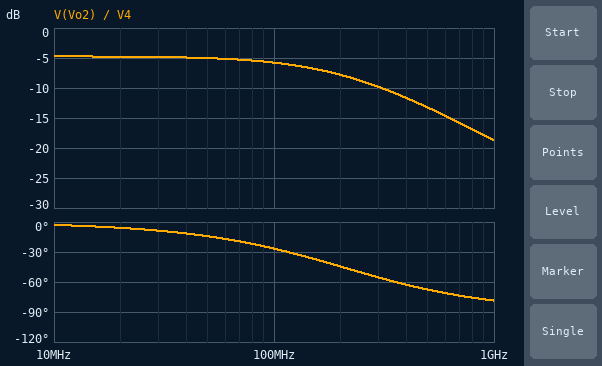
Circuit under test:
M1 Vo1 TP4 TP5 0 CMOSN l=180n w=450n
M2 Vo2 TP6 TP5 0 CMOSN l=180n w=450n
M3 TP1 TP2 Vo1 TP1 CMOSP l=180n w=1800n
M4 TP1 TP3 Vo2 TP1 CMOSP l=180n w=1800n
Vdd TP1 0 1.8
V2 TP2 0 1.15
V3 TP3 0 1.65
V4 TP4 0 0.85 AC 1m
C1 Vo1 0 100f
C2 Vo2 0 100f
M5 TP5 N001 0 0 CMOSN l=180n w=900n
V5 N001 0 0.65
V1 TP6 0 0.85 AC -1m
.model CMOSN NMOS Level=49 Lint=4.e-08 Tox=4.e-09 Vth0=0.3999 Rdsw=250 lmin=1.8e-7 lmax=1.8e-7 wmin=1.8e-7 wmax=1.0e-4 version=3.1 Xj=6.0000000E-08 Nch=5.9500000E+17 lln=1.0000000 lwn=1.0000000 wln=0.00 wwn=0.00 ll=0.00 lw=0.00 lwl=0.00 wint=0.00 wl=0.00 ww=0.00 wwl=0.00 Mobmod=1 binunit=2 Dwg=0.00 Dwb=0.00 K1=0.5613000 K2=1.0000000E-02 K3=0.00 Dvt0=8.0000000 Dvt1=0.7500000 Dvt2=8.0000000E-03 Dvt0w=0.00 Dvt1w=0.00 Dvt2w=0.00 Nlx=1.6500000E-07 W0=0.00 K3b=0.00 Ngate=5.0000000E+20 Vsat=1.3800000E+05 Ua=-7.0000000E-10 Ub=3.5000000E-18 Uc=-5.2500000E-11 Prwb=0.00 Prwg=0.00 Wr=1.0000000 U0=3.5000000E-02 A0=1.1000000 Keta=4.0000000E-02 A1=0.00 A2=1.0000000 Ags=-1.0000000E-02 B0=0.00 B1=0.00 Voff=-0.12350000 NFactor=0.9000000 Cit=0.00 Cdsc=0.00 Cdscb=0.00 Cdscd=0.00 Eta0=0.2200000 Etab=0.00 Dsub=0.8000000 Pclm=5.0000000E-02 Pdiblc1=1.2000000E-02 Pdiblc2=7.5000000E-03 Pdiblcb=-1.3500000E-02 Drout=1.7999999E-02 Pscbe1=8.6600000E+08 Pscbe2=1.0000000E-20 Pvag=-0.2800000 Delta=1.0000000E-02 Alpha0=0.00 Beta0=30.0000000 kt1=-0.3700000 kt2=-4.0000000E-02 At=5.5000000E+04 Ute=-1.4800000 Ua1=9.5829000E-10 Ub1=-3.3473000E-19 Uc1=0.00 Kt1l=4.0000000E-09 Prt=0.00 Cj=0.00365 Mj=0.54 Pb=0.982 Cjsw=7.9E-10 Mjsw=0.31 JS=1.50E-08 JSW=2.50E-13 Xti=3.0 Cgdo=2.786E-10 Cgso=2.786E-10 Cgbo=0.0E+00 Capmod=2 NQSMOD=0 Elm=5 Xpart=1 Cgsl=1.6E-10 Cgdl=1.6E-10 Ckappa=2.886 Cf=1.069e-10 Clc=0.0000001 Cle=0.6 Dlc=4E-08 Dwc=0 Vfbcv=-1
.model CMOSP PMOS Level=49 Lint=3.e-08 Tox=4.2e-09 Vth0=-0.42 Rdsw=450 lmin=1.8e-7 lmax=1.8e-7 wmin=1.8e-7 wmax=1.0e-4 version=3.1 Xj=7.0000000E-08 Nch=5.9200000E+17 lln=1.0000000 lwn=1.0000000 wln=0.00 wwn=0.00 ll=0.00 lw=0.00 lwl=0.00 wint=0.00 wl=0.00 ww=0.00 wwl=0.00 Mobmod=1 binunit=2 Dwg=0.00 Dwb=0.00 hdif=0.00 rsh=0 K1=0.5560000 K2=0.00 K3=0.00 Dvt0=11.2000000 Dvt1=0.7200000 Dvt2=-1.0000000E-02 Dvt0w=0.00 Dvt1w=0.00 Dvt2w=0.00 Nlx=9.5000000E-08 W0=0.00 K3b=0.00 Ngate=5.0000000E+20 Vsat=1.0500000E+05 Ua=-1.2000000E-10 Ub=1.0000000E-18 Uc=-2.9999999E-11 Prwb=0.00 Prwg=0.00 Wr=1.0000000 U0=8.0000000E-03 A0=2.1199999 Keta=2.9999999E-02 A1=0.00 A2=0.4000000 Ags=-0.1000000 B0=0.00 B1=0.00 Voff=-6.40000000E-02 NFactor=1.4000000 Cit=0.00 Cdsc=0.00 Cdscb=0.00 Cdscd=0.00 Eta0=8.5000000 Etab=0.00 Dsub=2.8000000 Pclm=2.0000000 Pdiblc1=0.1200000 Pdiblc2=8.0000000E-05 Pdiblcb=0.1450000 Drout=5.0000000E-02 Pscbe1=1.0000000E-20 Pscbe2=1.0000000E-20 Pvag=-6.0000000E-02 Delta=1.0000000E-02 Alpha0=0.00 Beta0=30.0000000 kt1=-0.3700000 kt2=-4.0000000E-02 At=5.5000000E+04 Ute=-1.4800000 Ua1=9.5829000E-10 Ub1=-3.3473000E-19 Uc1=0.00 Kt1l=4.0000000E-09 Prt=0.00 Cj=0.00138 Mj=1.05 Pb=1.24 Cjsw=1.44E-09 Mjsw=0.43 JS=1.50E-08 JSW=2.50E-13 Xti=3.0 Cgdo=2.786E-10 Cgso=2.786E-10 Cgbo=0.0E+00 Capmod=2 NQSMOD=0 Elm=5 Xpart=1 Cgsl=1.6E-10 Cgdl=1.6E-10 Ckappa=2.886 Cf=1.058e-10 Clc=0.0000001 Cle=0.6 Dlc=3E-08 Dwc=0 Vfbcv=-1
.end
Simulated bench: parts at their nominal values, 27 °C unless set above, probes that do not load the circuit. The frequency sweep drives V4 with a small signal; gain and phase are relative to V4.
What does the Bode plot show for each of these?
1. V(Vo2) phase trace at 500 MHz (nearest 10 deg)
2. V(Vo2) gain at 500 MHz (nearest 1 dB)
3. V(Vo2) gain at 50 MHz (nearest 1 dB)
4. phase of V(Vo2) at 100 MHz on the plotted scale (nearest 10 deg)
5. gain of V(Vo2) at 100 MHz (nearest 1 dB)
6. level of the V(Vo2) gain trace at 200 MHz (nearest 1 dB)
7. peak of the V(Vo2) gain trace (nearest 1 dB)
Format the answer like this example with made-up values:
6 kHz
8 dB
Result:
-70 deg
-13 dB
-5 dB
-30 deg
-6 dB
-8 dB
-5 dB
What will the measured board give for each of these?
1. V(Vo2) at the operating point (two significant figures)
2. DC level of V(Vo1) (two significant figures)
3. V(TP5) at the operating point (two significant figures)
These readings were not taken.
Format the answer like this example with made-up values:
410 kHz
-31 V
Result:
180 mV
1.6 V
180 mV
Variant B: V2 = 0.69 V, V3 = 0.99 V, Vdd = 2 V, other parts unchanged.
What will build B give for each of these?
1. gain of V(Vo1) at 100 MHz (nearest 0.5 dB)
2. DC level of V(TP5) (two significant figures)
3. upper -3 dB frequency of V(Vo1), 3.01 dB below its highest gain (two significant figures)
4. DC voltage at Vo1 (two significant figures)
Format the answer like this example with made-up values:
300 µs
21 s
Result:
-17.5 dB
280 mV
1.0 GHz
2.0 V
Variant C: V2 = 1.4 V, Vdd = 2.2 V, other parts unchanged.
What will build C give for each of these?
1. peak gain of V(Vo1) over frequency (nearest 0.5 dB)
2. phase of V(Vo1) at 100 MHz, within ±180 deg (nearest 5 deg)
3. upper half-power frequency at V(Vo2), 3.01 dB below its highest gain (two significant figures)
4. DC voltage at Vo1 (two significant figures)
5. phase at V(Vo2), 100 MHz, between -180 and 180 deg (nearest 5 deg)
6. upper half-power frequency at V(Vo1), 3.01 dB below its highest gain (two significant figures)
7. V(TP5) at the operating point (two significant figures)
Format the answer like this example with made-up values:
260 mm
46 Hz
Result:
-12.0 dB
170 deg
110 MHz
2.1 V
-40 deg
590 MHz
290 mV
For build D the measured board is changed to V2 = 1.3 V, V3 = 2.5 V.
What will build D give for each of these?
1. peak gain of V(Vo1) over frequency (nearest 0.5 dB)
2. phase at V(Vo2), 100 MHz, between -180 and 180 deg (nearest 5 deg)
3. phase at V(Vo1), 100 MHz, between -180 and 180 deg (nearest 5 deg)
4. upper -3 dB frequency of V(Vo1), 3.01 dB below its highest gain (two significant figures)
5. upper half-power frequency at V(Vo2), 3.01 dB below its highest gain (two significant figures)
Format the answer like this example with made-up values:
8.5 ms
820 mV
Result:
9.5 dB
-15 deg
120 deg
38 MHz
290 MHz
